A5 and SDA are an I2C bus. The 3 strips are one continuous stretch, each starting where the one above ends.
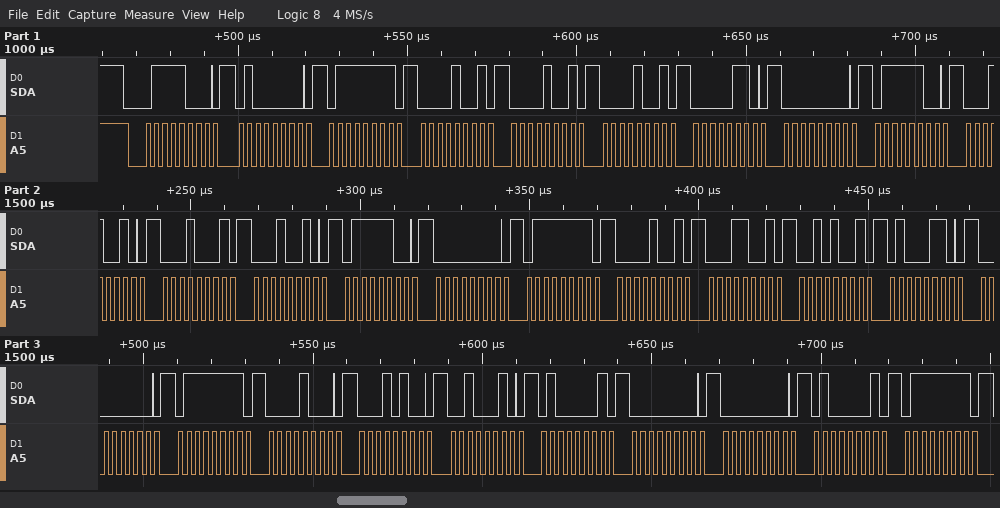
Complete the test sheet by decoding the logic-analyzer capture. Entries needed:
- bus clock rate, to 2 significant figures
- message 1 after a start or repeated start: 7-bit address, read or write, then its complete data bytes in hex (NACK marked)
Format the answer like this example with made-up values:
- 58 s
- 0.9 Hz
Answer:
- 400 kHz
- 0x3C write: 40 7F 09 09 09 06 00 7C 12 11 12 7C 00 7F 09 19 29 46 00 7F 08 14 22 41 00 00 41 7F
